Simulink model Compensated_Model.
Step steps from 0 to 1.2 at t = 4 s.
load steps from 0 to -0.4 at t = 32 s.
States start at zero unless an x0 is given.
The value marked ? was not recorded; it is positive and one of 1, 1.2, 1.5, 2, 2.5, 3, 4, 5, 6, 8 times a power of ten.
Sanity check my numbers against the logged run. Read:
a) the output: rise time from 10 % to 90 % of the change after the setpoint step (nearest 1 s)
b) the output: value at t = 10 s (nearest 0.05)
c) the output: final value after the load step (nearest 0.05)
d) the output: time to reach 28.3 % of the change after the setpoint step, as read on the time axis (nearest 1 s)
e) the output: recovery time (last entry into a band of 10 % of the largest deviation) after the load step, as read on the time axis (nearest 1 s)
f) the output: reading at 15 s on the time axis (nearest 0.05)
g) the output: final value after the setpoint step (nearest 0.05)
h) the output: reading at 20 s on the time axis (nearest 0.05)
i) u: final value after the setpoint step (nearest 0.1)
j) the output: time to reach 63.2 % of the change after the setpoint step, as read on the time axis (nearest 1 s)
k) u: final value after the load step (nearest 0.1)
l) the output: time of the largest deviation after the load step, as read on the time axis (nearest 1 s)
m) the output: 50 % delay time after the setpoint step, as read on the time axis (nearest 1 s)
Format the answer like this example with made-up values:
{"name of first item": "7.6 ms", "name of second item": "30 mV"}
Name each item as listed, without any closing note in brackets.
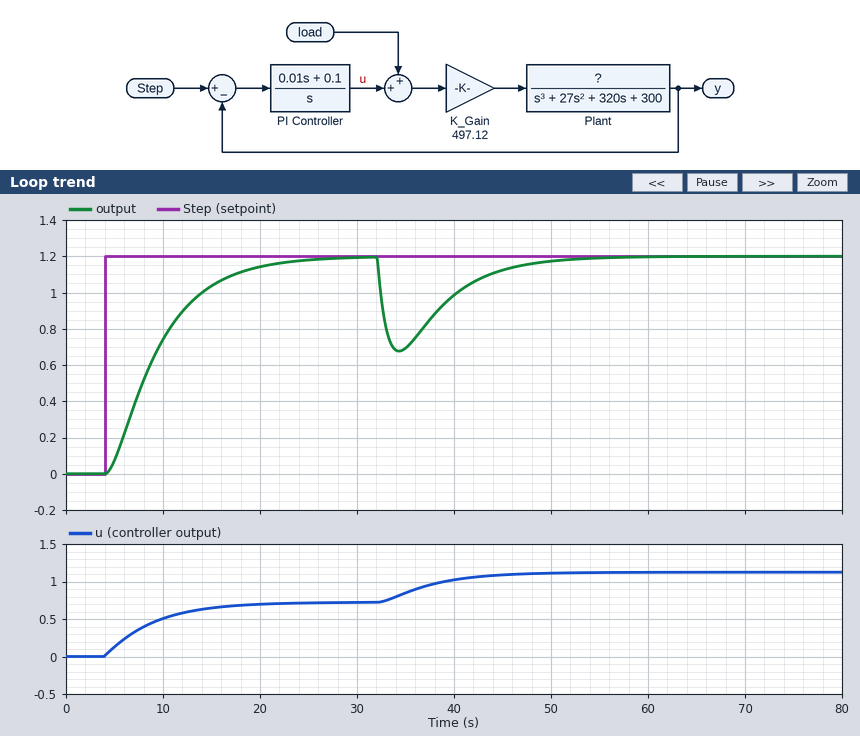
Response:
{"the output: rise time from 10 % to 90 % of the change after the setpoint step": "11 s", "the output: value at t = 10 s": "0.75", "the output: final value after the load step": "1.20", "the output: time to reach 28.3 % of the change after the setpoint step, as read on the time axis": "7 s", "the output: recovery time (last entry into a band of 10 % of the largest deviation) after the load step, as read on the time axis": "47 s", "the output: reading at 15 s on the time axis": "1.05", "the output: final value after the setpoint step": "1.20", "the output: reading at 20 s on the time axis": "1.15", "u: final value after the setpoint step": "0.7", "the output: time to reach 63.2 % of the change after the setpoint step, as read on the time axis": "10 s", "u: final value after the load step": "1.1", "the output: time of the largest deviation after the load step, as read on the time axis": "34 s", "the output: 50 % delay time after the setpoint step, as read on the time axis": "9 s"}
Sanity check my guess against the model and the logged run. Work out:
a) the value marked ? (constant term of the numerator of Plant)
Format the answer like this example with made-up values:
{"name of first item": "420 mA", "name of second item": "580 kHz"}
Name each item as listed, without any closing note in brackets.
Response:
{"the value marked ?": "1"}
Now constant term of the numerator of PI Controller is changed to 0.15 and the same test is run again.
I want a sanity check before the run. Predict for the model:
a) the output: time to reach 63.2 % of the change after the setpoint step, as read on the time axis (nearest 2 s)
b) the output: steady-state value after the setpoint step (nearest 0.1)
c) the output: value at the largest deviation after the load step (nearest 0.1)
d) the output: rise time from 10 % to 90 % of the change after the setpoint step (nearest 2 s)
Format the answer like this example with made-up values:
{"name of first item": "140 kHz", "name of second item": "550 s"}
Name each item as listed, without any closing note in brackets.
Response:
{"the output: time to reach 63.2 % of the change after the setpoint step, as read on the time axis": "8 s", "the output: steady-state value after the setpoint step": "1.2", "the output: value at the largest deviation after the load step": "0.7", "the output: rise time from 10 % to 90 % of the change after the setpoint step": "6 s"}
